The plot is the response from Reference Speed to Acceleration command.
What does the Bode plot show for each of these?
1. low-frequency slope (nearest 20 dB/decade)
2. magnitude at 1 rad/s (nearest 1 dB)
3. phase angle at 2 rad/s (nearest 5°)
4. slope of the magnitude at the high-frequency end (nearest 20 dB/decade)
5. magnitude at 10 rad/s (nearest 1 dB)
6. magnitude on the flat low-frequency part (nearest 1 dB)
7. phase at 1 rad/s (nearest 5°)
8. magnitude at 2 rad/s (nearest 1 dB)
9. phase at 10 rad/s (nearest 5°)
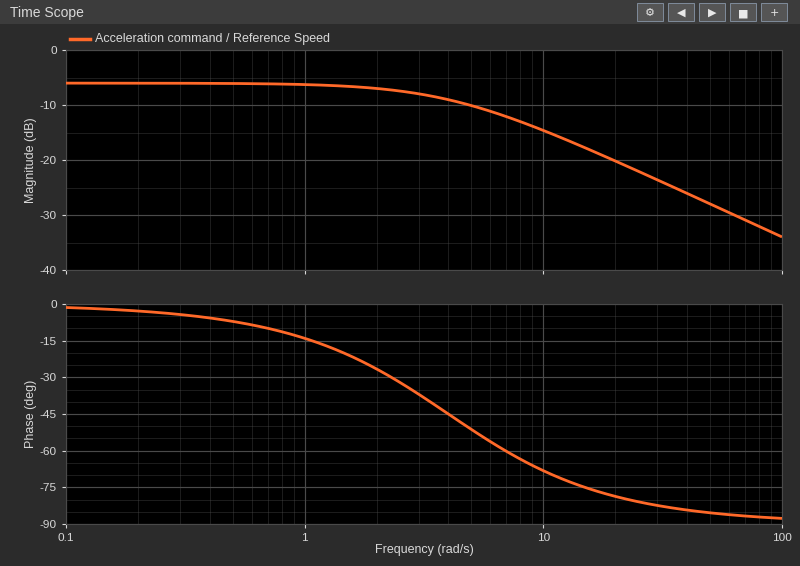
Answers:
0 dB/decade
-6 dB
-25°
-20 dB/decade
-15 dB
-6 dB
-15°
-7 dB
-70°
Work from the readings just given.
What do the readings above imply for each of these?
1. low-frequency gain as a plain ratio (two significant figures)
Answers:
0.50
